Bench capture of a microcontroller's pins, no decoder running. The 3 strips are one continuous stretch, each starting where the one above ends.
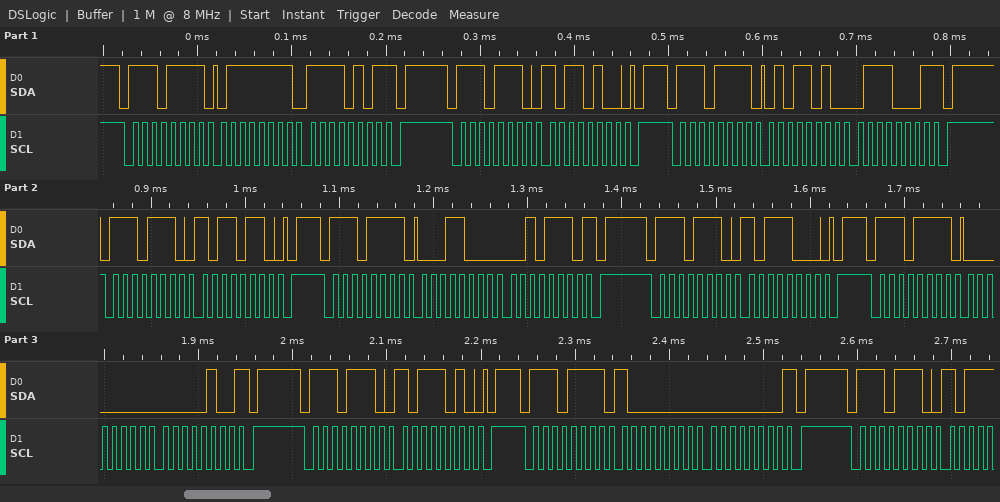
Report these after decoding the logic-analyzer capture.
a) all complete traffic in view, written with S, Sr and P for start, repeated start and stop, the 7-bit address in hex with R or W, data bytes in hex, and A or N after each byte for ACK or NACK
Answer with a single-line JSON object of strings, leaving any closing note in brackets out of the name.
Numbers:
{"all complete traffic in view, written with S, Sr and P for start, repeated start and stop, the 7-bit address in hex with R or W, data bytes in hex, and A or N after each byte for ACK or NACK": "S 77R A 7F A F5 N P S 77W A B4 A P S 77R A 5A A 71 N P S 77W A B6 A P S 77R A 18 A 2E N P S 77W A B8 A P S 77R A 00 A 04 N P S 77W A BA A P S 77R A 80 A 00 N P S 77W A"}
